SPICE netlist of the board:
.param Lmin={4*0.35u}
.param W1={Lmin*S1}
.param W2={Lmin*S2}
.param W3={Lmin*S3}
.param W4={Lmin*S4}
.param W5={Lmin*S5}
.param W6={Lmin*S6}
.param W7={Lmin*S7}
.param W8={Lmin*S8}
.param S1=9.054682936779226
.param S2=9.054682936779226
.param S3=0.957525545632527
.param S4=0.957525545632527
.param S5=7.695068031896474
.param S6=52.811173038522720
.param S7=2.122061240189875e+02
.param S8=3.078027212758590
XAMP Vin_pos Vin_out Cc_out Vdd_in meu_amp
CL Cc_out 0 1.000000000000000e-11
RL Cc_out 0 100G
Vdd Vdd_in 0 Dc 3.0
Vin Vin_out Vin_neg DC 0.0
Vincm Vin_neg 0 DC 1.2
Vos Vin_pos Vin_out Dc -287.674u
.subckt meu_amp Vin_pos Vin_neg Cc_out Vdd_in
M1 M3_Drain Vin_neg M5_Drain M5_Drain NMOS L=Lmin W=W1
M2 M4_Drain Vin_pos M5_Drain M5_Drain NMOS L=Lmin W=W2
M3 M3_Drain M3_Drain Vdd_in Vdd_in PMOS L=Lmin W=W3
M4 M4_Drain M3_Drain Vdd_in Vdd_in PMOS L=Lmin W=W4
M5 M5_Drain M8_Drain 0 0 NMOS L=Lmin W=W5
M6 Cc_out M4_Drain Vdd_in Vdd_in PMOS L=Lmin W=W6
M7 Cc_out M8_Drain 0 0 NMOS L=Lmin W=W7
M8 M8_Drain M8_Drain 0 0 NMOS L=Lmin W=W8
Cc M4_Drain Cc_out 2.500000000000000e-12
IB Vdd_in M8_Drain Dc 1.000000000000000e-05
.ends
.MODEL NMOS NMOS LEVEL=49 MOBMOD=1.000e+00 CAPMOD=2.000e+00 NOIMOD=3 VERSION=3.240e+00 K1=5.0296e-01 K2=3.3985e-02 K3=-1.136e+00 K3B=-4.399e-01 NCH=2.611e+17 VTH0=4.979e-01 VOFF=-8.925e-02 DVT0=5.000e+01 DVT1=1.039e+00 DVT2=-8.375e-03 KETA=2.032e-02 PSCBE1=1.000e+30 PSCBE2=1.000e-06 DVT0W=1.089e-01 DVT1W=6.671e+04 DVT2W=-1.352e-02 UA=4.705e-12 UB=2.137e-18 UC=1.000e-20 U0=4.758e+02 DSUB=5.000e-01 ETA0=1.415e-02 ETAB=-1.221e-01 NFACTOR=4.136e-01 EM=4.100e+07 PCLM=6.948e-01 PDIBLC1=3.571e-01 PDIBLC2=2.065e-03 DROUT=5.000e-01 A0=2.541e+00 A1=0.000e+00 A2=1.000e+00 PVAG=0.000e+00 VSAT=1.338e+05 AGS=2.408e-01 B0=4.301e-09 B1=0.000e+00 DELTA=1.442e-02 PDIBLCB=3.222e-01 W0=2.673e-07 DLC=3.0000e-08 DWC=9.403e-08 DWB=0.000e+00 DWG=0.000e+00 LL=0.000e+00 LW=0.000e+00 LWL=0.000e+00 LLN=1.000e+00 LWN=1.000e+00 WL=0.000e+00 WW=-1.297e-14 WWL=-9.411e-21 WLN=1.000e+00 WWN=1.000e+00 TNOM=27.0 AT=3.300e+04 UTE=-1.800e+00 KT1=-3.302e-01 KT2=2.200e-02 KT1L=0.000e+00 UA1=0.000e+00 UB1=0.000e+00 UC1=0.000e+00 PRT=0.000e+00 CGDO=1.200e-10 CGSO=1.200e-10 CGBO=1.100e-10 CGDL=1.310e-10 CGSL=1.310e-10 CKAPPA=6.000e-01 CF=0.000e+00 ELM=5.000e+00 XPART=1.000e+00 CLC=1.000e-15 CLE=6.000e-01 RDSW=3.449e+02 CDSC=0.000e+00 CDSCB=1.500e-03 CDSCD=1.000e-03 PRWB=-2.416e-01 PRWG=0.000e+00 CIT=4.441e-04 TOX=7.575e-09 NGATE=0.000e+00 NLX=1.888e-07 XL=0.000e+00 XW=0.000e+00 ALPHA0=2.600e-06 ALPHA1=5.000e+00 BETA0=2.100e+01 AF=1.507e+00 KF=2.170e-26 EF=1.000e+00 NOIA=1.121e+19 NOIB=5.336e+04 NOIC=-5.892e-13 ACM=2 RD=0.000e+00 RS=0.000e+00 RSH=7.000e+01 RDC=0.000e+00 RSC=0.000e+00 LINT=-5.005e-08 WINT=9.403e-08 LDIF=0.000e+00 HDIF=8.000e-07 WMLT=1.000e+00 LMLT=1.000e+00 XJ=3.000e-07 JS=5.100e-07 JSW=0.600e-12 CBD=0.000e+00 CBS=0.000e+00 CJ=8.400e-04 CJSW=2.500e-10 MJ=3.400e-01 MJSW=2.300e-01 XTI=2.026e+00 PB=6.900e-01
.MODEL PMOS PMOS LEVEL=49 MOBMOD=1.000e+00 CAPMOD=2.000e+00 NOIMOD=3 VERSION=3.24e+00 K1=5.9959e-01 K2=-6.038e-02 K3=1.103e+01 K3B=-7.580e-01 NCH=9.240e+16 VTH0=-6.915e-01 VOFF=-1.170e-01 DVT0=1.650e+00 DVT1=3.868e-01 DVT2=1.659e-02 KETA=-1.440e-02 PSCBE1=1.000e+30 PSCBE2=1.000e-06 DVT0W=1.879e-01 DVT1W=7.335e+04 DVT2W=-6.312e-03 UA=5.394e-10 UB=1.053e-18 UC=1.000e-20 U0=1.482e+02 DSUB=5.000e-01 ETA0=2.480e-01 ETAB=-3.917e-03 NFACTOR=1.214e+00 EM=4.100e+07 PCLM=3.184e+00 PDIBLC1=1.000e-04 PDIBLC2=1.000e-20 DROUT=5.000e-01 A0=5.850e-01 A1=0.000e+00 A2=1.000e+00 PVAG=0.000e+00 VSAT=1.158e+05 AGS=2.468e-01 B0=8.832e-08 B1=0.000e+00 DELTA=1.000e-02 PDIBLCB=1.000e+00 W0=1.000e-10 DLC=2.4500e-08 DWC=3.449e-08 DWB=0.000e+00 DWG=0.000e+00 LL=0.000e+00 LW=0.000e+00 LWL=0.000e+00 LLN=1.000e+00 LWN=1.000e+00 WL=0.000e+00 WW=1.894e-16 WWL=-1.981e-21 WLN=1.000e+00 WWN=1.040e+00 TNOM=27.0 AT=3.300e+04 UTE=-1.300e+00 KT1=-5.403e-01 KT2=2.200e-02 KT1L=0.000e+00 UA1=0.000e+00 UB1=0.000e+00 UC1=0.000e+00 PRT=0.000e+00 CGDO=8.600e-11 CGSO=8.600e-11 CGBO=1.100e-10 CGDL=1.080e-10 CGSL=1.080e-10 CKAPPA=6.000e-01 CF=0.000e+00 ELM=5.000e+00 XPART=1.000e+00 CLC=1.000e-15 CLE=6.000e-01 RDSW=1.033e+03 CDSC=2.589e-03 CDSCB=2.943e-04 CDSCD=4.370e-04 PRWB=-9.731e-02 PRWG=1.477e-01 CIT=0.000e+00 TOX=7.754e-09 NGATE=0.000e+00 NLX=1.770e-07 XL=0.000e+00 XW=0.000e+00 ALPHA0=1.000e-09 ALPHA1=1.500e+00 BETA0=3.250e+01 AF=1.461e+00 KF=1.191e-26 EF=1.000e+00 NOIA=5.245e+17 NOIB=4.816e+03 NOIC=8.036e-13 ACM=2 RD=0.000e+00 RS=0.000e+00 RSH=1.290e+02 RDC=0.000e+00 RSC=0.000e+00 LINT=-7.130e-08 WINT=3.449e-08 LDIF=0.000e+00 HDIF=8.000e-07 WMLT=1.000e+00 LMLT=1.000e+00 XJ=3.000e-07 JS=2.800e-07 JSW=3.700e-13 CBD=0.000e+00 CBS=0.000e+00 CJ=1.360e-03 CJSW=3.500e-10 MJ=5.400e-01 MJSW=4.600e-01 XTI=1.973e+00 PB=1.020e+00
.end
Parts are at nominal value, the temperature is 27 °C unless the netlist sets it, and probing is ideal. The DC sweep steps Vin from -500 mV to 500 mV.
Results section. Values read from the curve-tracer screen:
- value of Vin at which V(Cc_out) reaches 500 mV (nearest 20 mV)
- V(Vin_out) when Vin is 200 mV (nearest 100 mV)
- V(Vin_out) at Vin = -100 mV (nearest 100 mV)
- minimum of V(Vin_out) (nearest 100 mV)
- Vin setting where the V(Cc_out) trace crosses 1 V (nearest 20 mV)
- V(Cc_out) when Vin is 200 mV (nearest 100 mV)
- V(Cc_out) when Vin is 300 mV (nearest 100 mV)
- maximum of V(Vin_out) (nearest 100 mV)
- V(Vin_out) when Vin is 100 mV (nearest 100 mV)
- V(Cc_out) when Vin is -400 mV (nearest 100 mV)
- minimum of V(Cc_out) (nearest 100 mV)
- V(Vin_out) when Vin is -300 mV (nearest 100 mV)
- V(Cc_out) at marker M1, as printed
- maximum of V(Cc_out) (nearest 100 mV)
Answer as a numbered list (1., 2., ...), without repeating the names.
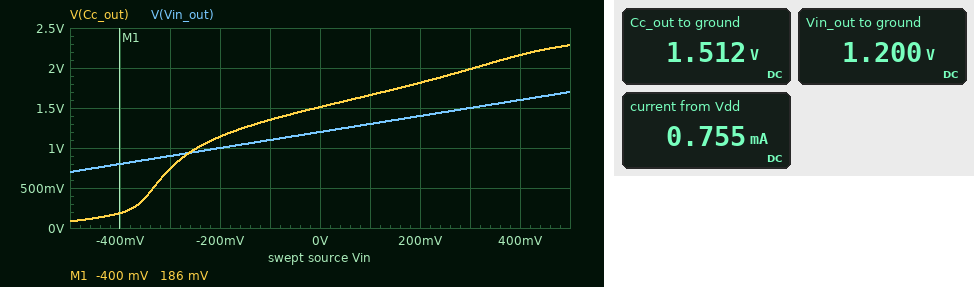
1. -340 mV
2. 1.4 V
3. 1.1 V
4. 700 mV
5. -240 mV
6. 1.8 V
7. 2.0 V
8. 1.7 V
9. 1.3 V
10. 200 mV
11. 100 mV
12. 900 mV
13. 186 mV
14. 2.3 V
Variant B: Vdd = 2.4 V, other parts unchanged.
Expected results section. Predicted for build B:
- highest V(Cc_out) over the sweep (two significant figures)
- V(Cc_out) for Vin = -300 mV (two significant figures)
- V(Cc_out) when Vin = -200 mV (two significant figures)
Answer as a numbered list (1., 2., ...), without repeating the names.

1. 1.8 V
2. 880 mV
3. 1.4 V
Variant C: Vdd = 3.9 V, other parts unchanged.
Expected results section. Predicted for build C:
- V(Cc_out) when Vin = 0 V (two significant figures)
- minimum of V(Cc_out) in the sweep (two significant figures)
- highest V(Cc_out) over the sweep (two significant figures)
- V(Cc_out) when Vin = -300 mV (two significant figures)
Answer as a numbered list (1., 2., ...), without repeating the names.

1. 1.8 V
2. 88 mV
3. 2.2 V
4. 1.2 V
